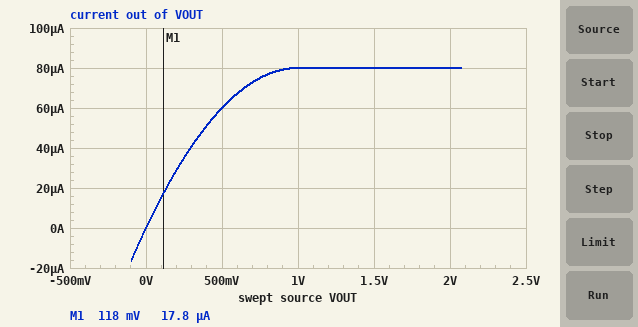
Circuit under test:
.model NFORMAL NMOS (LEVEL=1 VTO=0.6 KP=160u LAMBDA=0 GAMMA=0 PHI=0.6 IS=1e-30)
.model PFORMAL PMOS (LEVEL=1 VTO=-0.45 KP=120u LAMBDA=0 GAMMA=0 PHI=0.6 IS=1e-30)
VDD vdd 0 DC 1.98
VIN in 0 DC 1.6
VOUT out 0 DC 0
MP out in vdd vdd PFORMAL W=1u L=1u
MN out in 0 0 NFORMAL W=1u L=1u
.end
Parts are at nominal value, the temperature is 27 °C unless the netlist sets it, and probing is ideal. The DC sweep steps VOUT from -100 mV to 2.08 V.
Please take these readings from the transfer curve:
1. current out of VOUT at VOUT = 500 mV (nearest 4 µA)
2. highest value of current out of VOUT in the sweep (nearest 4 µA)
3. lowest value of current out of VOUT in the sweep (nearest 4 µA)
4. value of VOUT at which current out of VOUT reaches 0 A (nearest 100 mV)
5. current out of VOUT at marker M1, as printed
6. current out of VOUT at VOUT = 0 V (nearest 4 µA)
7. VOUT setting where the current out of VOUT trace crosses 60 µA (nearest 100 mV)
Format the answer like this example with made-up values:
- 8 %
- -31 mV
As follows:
- 60 µA
- 80 µA
- -16 µA
- 0 V
- 17.8 µA
- 0 A
- 500 mV
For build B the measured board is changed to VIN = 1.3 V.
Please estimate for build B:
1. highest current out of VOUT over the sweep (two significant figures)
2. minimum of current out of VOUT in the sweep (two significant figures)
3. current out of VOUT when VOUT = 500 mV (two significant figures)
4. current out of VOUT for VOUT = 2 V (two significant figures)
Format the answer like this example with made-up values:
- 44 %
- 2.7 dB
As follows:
- 43 µA
- -15 µA
- 33 µA
- 40 µA
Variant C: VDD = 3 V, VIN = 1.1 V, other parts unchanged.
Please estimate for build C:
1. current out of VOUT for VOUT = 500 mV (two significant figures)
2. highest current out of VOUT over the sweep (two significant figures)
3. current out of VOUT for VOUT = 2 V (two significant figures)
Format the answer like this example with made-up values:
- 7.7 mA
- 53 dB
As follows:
- -110 µA
- -89 µA
- -94 µA
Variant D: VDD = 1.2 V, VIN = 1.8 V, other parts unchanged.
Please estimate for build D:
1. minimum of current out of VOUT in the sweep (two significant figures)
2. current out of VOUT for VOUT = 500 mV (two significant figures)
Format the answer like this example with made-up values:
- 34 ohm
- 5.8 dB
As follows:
- -20 µA
- 76 µA
